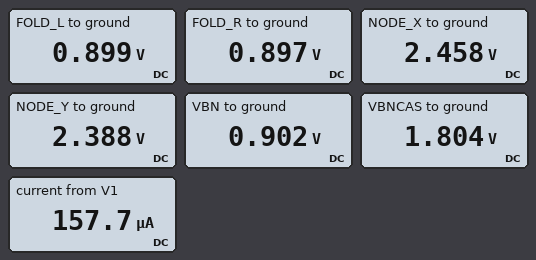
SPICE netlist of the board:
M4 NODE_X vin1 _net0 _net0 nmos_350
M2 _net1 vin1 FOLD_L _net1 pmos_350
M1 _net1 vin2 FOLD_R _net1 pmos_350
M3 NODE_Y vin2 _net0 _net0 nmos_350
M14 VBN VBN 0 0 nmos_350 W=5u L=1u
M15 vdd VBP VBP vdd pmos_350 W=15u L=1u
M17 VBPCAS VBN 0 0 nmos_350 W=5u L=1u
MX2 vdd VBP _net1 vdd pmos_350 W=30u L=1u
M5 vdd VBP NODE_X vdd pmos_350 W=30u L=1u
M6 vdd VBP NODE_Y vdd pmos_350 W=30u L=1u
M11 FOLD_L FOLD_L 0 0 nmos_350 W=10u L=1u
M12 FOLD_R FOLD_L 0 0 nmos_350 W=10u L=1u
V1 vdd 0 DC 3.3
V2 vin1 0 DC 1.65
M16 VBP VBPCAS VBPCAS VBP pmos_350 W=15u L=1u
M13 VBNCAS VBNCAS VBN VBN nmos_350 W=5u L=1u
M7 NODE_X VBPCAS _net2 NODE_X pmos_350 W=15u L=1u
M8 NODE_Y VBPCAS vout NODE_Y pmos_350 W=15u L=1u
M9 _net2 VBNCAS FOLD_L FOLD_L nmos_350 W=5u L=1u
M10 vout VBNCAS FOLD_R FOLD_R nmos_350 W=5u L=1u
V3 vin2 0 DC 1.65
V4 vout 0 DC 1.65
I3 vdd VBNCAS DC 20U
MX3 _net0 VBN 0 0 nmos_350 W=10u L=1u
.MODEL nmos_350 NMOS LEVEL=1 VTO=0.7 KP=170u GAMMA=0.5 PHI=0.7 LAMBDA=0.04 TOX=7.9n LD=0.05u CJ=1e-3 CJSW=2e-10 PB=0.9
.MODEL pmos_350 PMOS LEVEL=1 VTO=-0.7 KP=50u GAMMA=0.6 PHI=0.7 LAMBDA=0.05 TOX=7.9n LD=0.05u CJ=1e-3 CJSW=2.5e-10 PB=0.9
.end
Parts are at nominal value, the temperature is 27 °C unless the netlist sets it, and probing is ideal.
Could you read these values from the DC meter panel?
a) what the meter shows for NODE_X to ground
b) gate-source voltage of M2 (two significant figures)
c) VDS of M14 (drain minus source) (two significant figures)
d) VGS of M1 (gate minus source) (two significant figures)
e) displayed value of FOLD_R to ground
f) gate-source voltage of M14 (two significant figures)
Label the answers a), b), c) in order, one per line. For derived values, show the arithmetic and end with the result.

a) 2.458 V
b) 1.65 V - 899 mV = 750 mV
c) 902 mV = 900 mV
d) 1.65 V - 897 mV = 750 mV
e) 0.897 V
f) 902 mV = 900 mV
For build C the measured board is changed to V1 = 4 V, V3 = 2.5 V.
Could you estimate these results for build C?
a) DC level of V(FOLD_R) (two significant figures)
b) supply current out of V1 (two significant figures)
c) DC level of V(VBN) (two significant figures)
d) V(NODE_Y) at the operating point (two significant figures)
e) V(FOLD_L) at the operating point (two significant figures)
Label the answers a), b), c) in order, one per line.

a) 780 mV
b) 140 µA
c) 900 mV
d) 2.9 V
e) 930 mV
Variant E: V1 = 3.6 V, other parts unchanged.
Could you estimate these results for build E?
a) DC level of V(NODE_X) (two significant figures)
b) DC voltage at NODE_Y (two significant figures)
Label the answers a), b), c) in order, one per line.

a) 3.1 V
b) 2.7 V
